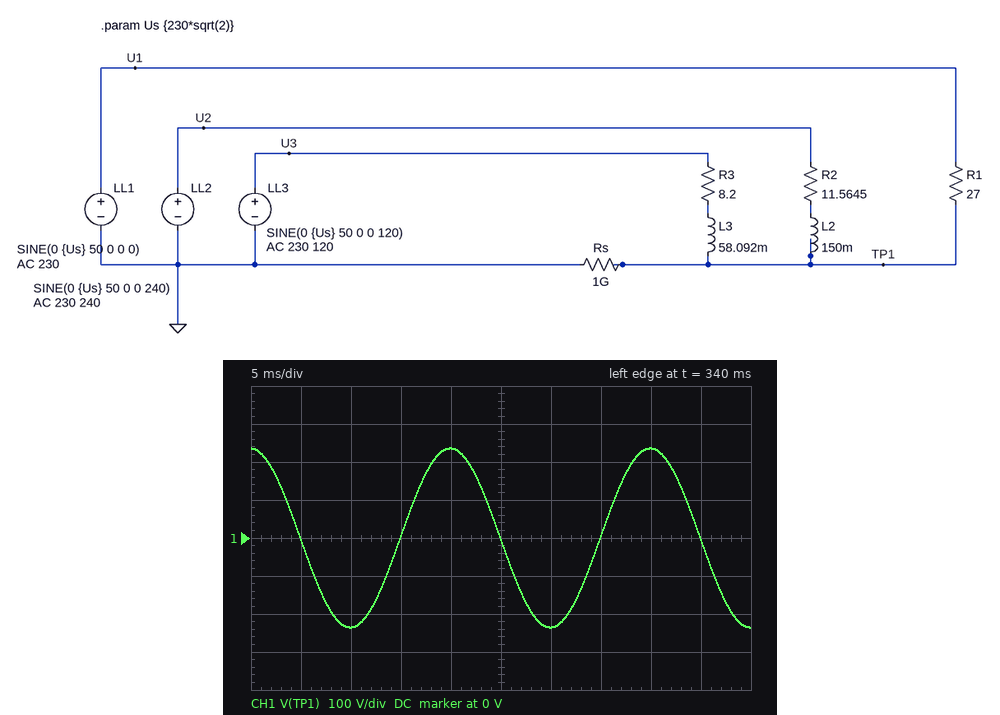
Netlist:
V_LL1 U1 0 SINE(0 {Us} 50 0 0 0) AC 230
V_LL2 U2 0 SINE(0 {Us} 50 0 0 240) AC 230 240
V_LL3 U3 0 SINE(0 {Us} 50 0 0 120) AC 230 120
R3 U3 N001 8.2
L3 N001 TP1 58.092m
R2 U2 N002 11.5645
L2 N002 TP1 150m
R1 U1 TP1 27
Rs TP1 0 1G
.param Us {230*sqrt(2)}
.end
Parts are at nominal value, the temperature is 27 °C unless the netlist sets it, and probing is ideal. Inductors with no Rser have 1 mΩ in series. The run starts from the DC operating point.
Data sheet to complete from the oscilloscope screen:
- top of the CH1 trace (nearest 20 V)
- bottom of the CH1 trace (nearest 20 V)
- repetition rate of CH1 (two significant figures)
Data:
240 V
-240 V
50 Hz
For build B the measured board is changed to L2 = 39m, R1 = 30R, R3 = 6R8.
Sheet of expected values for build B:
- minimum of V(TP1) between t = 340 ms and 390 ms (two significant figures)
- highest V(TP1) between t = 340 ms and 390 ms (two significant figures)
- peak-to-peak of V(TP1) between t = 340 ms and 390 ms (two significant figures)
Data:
-68 V
68 V
140 V
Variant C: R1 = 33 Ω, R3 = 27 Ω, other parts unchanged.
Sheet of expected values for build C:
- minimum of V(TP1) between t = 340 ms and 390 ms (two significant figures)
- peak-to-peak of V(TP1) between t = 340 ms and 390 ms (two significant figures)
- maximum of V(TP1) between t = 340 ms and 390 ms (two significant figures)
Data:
-180 V
350 V
180 V
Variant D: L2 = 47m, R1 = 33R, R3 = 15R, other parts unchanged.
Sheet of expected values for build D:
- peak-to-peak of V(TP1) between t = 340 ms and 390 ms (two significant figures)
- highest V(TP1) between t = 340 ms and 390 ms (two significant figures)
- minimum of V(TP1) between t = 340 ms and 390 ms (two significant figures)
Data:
180 V
92 V
-92 V
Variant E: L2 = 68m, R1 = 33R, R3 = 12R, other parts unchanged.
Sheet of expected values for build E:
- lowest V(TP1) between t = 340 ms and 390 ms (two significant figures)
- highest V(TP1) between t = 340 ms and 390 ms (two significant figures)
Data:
-130 V
130 V
